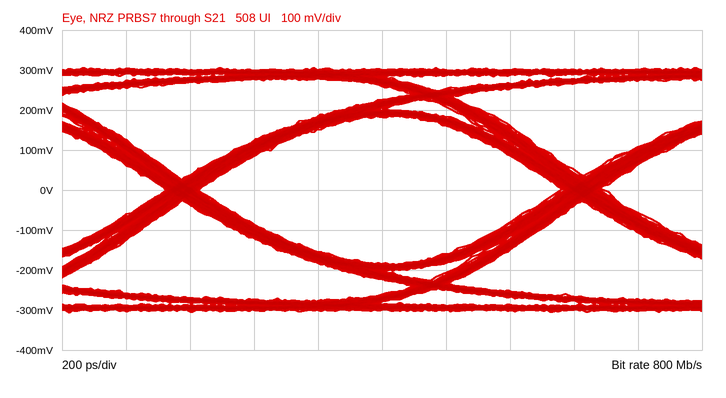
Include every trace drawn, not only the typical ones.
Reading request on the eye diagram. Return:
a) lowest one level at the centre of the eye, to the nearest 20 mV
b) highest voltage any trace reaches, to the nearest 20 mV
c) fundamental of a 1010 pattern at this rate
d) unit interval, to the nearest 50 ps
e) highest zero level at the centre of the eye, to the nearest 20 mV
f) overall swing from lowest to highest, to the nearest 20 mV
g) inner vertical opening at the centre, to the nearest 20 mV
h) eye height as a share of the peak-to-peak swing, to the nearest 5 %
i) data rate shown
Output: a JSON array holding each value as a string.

["180 mV", "300 mV", "400 MHz", "1.25 ns", "-180 mV", "620 mV", "360 mV", "60 %", "800 Mb/s"]
